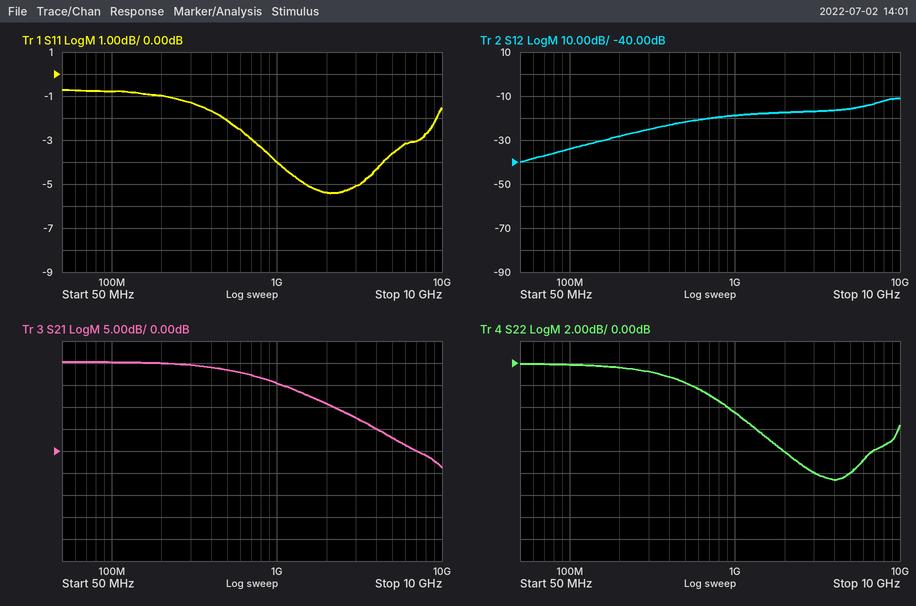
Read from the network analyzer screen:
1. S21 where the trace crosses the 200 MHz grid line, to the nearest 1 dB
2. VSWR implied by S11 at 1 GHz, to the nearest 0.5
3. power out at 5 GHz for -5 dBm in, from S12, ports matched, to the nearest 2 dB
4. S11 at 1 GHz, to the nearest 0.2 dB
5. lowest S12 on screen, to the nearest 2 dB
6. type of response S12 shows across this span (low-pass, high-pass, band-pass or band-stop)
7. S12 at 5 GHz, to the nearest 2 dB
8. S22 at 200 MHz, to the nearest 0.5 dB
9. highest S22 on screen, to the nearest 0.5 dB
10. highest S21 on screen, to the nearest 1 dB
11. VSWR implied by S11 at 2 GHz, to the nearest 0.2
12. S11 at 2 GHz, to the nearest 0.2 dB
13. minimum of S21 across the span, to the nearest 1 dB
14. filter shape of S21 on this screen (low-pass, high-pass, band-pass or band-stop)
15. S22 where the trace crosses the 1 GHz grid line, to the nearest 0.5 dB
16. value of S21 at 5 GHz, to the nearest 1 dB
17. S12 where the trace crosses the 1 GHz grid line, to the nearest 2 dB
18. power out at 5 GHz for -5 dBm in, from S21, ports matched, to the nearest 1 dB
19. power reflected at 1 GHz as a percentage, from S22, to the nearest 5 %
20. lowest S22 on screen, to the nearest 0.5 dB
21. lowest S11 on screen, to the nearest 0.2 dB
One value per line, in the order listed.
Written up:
20 dB
4.5
-20 dBm
-4.0 dB
-40 dB
high-pass
-16 dB
-0.5 dB
0.0 dB
20 dB
3.4
-5.4 dB
-4 dB
low-pass
-4.5 dB
3 dB
-18 dB
-2 dBm
35 %
-10.5 dB
-5.4 dB
